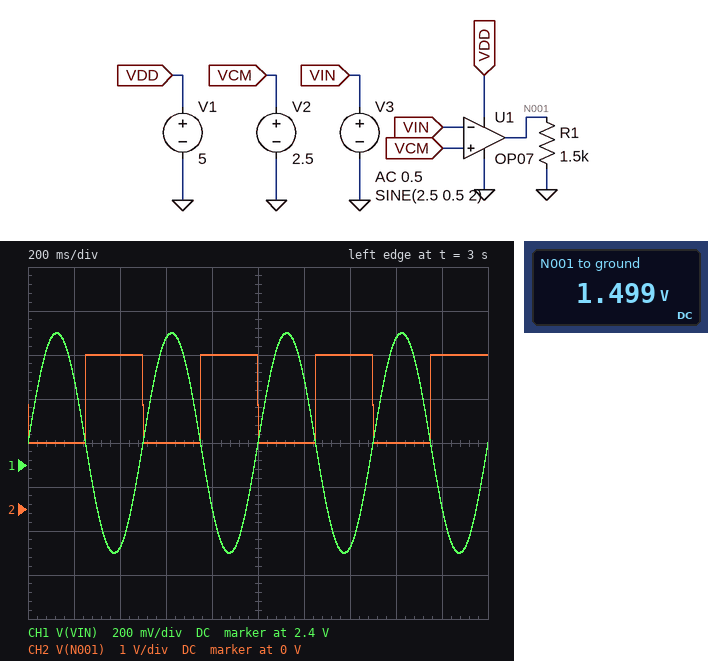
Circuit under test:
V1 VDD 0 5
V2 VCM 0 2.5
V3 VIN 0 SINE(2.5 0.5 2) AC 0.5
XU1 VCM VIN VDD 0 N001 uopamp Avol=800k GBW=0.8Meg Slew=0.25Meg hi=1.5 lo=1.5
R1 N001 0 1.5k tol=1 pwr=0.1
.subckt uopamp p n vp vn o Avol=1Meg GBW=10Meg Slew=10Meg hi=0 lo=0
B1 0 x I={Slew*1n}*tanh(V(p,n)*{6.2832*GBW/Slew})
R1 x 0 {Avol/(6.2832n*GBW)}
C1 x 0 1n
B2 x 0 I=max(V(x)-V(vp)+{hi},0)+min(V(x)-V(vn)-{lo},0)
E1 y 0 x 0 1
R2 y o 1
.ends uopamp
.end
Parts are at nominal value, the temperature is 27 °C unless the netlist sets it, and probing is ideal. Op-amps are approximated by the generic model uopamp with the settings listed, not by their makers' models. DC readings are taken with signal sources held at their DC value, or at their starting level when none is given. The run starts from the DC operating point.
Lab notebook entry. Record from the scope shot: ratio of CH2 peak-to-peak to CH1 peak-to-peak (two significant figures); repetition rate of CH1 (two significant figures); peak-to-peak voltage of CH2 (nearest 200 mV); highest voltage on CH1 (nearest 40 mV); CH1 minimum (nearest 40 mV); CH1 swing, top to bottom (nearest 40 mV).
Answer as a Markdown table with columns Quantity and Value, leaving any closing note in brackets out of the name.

| Quantity | Value |
|---|---|
| ratio of CH2 peak-to-peak to CH1 peak-to-peak | 2.0 |
| repetition rate of CH1 | 2.0 Hz |
| peak-to-peak voltage of CH2 | 2.0 V |
| highest voltage on CH1 | 3.00 V |
| CH1 minimum | 2.00 V |
| CH1 swing, top to bottom | 1.00 V |
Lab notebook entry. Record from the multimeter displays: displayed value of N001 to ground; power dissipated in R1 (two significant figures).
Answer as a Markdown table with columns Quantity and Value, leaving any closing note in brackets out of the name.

| Quantity | Value |
|---|---|
| displayed value of N001 to ground | 1.499 V |
| power dissipated in R1 | 1.5 mW |
